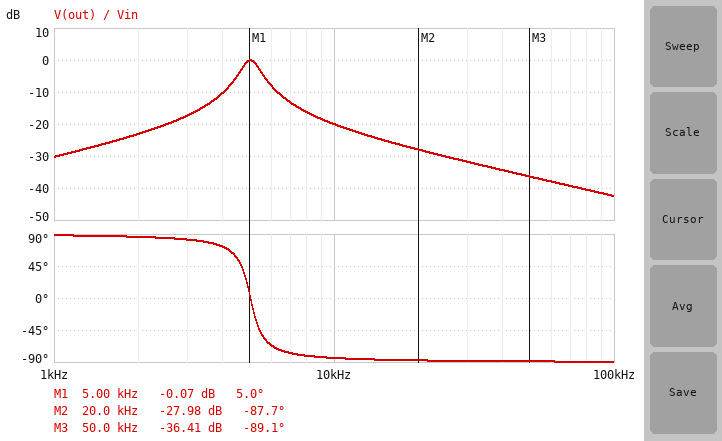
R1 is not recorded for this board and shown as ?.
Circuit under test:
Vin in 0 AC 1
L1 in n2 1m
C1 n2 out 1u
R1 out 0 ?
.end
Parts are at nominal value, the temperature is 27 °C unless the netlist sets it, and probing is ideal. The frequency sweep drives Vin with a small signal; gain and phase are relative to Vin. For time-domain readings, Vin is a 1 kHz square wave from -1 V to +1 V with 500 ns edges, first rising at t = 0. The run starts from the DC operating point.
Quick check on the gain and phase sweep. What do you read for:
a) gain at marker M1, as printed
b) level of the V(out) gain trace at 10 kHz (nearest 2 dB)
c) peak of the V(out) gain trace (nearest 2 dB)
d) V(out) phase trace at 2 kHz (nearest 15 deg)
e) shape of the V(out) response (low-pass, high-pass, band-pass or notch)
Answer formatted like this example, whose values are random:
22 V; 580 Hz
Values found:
-0.07 dB; -20 dB; 0 dB; 90 deg; band-pass
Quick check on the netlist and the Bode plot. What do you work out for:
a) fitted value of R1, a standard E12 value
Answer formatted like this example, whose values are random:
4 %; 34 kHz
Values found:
4.7 Ω
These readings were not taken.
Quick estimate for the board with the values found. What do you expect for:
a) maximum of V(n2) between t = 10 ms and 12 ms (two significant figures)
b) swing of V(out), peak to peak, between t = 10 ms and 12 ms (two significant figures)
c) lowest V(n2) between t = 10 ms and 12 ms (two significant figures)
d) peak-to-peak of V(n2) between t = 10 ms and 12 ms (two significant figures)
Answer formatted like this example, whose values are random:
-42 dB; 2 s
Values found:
3.3 V; 770 mV; -3.3 V; 6.6 V
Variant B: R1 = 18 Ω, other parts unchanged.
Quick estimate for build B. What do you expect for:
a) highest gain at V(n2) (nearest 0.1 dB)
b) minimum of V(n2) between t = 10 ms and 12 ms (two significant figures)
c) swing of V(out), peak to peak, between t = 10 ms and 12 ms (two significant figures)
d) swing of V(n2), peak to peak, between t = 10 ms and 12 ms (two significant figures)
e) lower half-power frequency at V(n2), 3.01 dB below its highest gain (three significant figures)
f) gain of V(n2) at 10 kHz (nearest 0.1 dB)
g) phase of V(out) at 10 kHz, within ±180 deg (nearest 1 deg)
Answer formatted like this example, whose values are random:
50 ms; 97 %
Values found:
6.3 dB; -1.9 V; 1.6 V; 3.9 V; 3.04 kHz; -6.4 dB; -69 deg
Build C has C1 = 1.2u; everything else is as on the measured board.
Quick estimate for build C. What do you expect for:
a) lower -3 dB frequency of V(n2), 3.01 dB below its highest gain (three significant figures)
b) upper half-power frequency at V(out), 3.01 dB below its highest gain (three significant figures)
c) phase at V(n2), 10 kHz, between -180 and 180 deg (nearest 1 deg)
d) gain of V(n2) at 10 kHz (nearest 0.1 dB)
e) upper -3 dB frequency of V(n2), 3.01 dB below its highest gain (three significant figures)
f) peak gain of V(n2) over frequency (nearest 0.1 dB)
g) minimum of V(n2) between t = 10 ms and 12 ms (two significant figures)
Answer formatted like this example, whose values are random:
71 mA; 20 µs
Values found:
4.17 kHz; 4.98 kHz; -155 deg; -11.0 dB; 4.93 kHz; 15.9 dB; -2.6 V
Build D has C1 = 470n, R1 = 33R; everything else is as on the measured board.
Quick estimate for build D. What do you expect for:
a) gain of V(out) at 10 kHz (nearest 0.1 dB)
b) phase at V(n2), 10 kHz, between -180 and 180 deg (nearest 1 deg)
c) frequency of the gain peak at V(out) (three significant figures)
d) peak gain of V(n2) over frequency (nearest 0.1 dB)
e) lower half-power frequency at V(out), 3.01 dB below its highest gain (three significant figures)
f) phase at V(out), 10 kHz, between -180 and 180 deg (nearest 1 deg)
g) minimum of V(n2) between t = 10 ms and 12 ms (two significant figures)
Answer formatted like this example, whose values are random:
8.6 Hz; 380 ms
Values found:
-2.5 dB; -87 deg; 7.34 kHz; 5.0 dB; 5.17 kHz; -41 deg; -1.8 V
